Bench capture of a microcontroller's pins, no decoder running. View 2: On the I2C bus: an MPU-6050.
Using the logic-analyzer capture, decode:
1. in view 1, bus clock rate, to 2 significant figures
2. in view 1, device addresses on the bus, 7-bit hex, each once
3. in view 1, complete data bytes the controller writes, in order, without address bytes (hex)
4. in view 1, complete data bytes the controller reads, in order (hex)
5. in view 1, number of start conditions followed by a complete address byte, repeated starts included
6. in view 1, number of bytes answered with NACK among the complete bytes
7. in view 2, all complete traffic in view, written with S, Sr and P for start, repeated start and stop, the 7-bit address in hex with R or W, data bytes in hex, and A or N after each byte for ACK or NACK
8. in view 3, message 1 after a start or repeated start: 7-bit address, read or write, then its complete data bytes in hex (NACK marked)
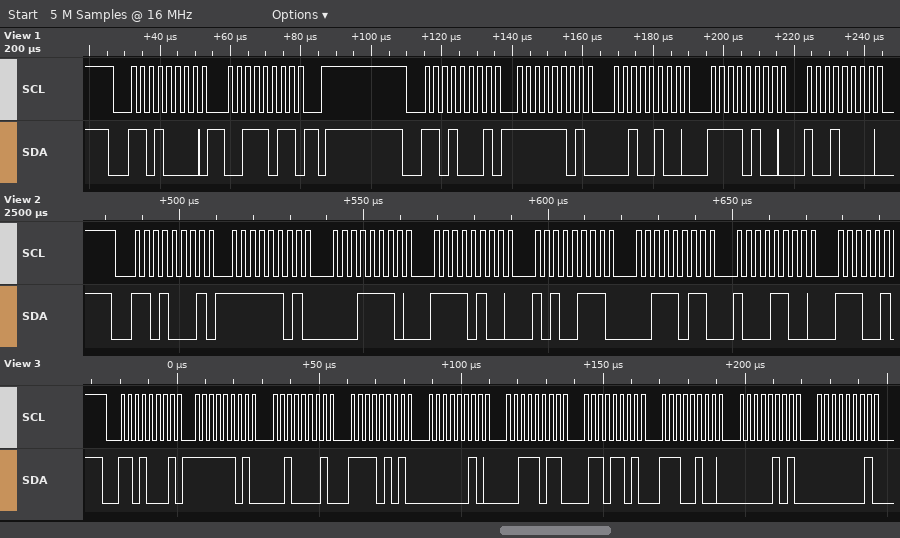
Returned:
400 kHz
0x68
3B
FD 24 F4 90
2
0
S 68R A FD A 1E A F4 A A7 A 3B A 8C A
0x68 read: FD 21 F5 02 3B 6D E4 05 01
